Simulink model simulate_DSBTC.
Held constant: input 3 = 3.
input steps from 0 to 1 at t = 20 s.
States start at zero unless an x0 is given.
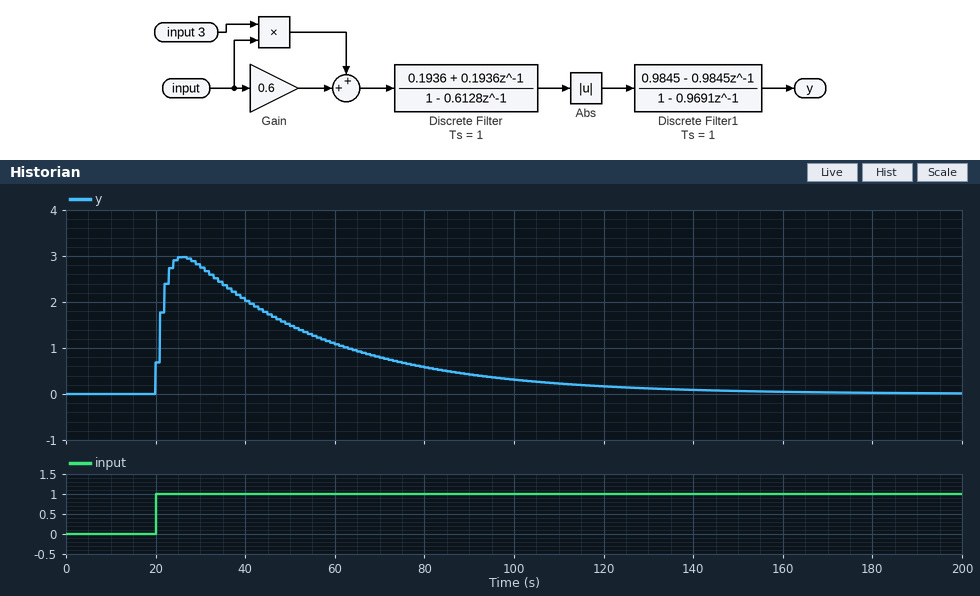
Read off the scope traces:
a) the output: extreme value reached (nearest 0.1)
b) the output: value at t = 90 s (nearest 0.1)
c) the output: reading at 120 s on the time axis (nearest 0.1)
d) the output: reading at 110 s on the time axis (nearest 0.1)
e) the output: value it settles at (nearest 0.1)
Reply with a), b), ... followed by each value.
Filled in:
a) 3.0
b) 0.4
c) 0.2
d) 0.2
e) 0.0
